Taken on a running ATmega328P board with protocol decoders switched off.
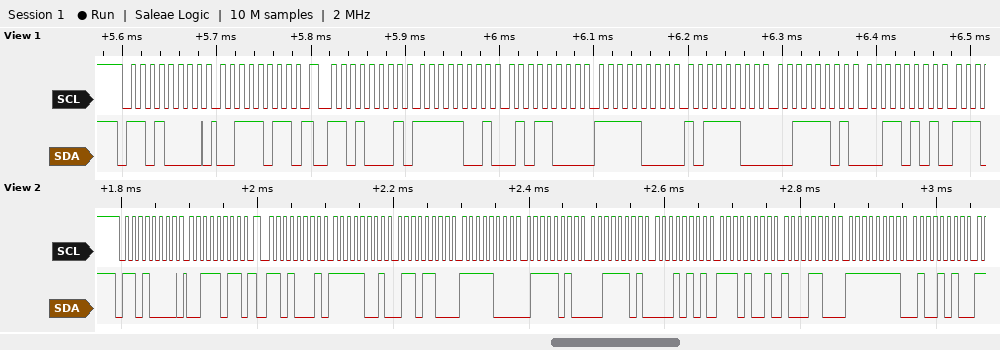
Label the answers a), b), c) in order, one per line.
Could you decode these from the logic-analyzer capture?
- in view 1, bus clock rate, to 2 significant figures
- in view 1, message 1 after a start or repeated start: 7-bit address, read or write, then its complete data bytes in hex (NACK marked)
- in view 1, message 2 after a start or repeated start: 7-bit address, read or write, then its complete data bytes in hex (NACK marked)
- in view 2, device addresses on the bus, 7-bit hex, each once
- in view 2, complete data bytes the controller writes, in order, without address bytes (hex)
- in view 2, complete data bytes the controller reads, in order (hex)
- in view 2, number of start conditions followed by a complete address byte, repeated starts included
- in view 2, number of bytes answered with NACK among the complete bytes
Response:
a) 100 kHz
b) 0x68 write: 3B
c) 0x68 read: F9 58 F8 BC 3D 35
d) 0x68
e) 3B
f) F9 6C F8 7A 3D 15 E9 8C FF 4A
g) 2
h) 0
